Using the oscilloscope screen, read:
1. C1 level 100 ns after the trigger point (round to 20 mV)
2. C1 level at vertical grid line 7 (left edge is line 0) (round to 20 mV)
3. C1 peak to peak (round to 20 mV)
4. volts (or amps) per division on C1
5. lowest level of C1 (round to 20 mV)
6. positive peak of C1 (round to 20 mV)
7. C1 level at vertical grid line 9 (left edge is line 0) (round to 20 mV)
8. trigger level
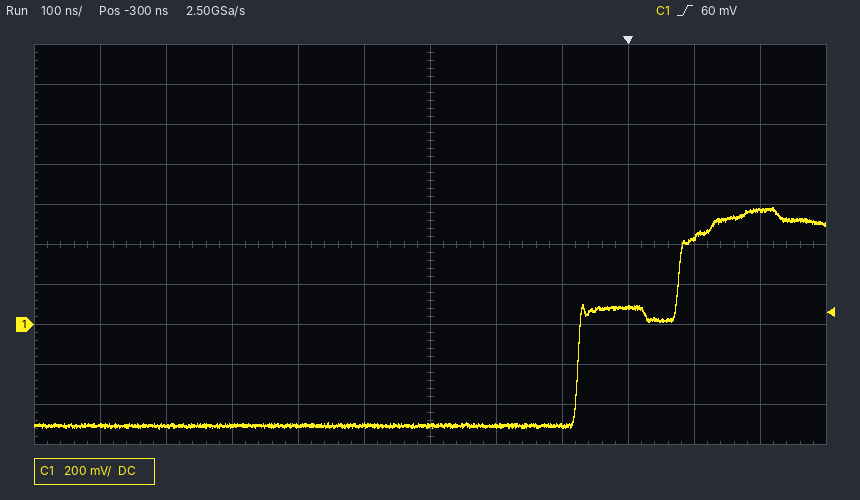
440 mV
-500 mV
1.10 V
200 mV
-520 mV
580 mV
80 mV
60 mV
